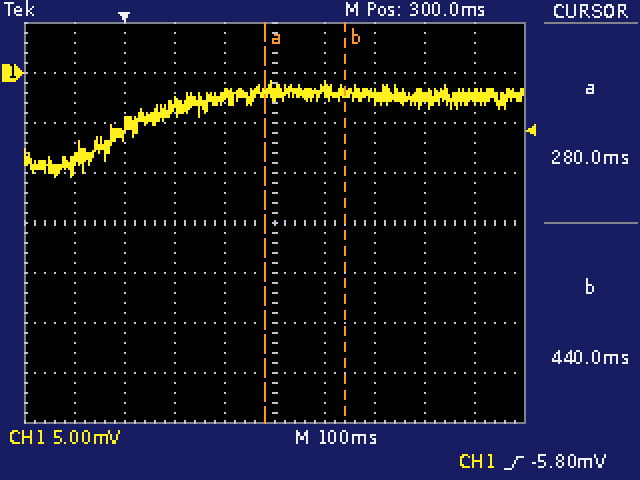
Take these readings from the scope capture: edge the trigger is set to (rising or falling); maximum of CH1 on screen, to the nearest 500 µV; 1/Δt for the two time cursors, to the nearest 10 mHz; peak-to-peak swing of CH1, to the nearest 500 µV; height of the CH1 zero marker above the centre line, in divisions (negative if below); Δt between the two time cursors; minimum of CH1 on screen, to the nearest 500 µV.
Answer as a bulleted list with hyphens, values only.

- rising
- -1.0 mV
- 6.25 Hz
- 9.5 mV
- +3.0 div
- 160 ms
- -10.5 mV
